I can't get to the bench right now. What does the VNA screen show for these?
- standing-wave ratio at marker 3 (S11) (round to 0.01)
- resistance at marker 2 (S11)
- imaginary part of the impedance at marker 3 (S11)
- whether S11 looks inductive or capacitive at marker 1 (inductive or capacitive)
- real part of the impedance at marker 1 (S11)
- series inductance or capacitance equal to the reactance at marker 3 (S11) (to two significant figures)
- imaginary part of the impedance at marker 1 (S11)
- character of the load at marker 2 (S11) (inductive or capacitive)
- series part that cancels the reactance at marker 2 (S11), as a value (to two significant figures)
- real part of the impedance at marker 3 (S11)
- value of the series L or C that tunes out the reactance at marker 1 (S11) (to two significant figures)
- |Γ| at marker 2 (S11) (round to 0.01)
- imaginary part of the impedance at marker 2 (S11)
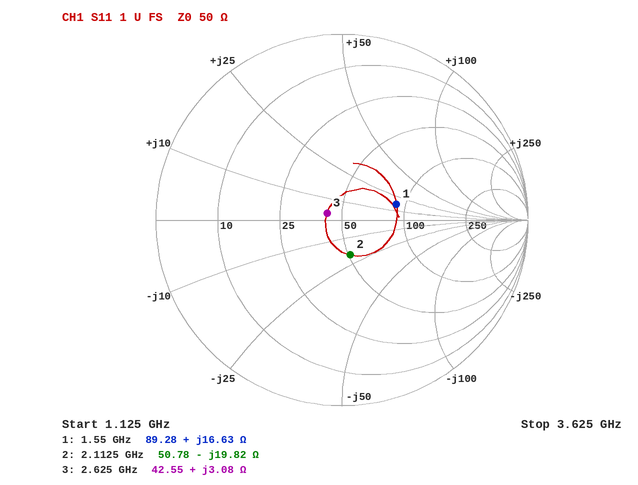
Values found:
1.19
50.78 Ω
+3.08 Ω
inductive
89.28 Ω
190 pH
+16.63 Ω
capacitive
1.5 nH
42.55 Ω
6.2 pF
0.19
-19.82 Ω
